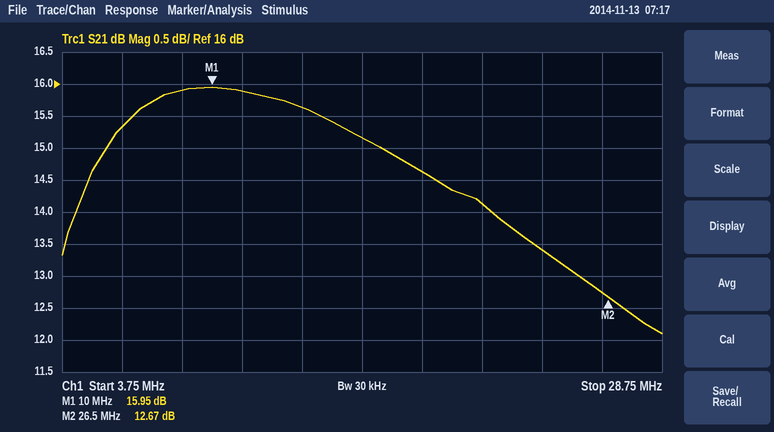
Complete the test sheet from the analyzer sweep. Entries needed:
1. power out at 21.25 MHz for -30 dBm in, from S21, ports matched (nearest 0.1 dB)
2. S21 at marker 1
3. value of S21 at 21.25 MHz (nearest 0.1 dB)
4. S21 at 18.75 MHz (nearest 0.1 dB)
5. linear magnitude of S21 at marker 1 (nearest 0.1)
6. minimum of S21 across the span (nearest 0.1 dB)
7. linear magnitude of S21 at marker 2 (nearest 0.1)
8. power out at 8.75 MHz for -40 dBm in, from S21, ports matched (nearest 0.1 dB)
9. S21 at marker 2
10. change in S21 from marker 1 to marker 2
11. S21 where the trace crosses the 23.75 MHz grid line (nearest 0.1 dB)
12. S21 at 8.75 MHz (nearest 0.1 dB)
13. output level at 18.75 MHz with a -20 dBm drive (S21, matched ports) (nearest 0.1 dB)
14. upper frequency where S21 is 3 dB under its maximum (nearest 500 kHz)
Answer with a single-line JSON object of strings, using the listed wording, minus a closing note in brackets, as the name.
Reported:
{"power out at 21.25 MHz for -30 dBm in, from S21, ports matched": "-15.9 dBm", "S21 at marker 1": "15.95 dB", "value of S21 at 21.25 MHz": "14.1 dB", "S21 at 18.75 MHz": "14.6 dB", "linear magnitude of S21 at marker 1": "6.3", "minimum of S21 across the span": "12.1 dB", "linear magnitude of S21 at marker 2": "4.3", "power out at 8.75 MHz for -40 dBm in, from S21, ports matched": "-24.1 dBm", "S21 at marker 2": "12.67 dB", "change in S21 from marker 1 to marker 2": "-3.28 dB", "S21 where the trace crosses the 23.75 MHz grid line": "13.4 dB", "S21 at 8.75 MHz": "15.9 dB", "output level at 18.75 MHz with a -20 dBm drive (S21, matched ports)": "-5.4 dBm", "upper frequency where S21 is 3 dB under its maximum": "25.5 MHz"}
